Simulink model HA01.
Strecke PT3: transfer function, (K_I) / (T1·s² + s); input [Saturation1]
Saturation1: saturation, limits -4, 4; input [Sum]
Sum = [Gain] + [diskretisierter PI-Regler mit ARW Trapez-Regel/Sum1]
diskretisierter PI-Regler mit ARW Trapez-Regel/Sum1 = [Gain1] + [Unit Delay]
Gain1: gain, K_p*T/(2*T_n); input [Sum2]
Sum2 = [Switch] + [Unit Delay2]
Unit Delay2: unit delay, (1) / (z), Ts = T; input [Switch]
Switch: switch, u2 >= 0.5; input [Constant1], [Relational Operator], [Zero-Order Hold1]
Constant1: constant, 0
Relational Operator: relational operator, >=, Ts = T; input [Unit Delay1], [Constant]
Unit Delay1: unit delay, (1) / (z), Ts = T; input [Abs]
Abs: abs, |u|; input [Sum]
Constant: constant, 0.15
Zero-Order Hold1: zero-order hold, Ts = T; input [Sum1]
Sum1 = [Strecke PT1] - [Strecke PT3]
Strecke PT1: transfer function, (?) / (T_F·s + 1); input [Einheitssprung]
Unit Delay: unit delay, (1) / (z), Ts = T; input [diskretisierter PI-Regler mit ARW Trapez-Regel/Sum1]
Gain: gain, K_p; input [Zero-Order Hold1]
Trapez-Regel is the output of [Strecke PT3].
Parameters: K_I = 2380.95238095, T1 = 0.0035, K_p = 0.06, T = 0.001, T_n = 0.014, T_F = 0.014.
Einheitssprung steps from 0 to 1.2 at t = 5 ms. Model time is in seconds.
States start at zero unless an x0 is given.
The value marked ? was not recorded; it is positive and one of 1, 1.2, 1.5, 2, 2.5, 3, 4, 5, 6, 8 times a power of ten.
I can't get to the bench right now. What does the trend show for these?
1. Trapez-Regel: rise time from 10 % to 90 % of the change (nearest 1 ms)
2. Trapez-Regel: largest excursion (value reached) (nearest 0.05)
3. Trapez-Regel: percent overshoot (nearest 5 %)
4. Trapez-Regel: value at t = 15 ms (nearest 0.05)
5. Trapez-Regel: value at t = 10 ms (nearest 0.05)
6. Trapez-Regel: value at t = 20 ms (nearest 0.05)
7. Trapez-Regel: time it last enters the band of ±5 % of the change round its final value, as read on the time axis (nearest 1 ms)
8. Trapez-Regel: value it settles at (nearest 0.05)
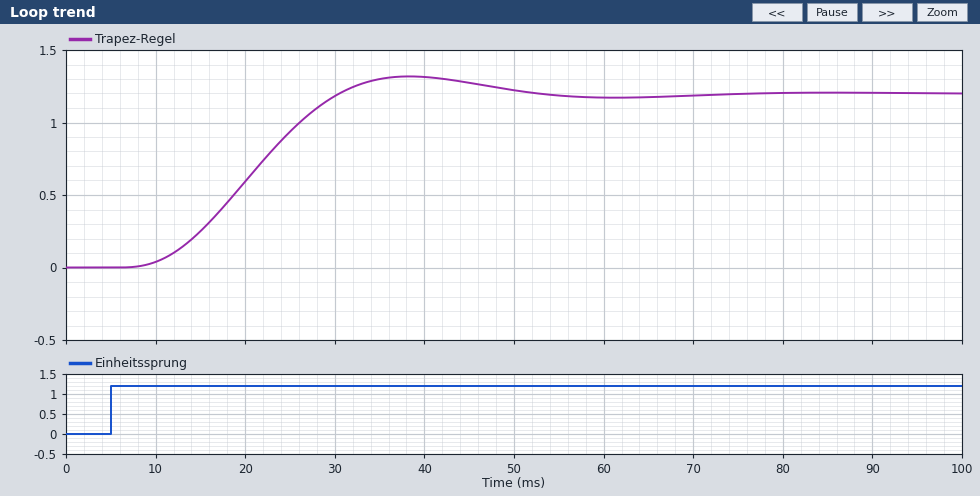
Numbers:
15 ms
1.30
10 %
0.25
0.05
0.60
46 ms
1.20
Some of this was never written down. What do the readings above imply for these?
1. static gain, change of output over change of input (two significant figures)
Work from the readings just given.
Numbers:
1.0
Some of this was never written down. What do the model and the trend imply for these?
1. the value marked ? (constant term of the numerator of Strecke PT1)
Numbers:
1
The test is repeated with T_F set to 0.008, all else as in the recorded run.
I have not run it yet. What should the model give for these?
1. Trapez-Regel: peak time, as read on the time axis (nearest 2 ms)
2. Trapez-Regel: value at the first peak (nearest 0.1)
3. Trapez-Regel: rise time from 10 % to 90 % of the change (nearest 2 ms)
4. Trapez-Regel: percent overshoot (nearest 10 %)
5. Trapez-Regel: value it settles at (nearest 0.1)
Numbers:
34 ms
1.5
12 ms
30 %
1.2
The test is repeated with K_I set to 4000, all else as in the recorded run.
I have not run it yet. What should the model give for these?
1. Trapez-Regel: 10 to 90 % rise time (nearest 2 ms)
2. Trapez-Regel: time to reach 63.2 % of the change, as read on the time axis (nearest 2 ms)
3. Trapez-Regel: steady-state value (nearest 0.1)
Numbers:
14 ms
20 ms
1.2
